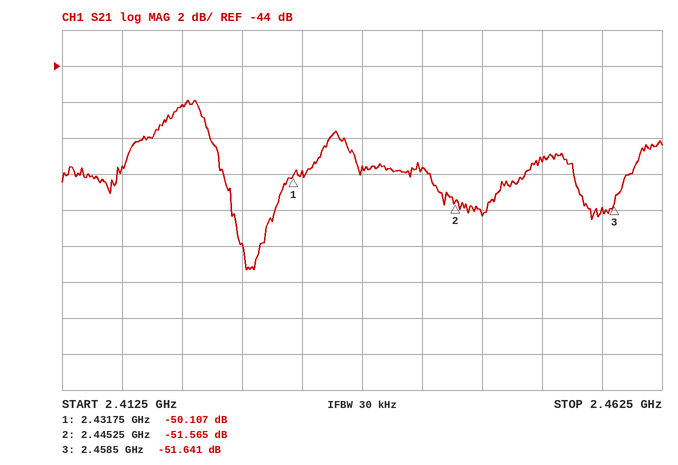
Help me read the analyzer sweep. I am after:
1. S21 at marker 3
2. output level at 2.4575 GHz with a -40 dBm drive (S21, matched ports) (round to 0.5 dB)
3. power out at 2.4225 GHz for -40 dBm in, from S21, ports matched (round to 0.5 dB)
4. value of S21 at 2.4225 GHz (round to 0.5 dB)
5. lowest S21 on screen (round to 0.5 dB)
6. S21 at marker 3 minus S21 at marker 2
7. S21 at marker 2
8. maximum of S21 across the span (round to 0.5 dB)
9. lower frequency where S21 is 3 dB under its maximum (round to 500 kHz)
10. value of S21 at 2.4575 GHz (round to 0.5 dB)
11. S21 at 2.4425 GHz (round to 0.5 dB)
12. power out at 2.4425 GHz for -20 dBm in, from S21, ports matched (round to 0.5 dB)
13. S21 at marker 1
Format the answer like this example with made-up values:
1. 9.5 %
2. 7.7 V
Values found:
1. -51.641 dB
2. -92.0 dBm
3. -86.0 dBm
4. -46.0 dB
5. -55.5 dB
6. -0.076 dB
7. -51.565 dB
8. -46.0 dB
9. 2.4180 GHz
10. -52.0 dB
11. -49.5 dB
12. -69.5 dBm
13. -50.107 dB
